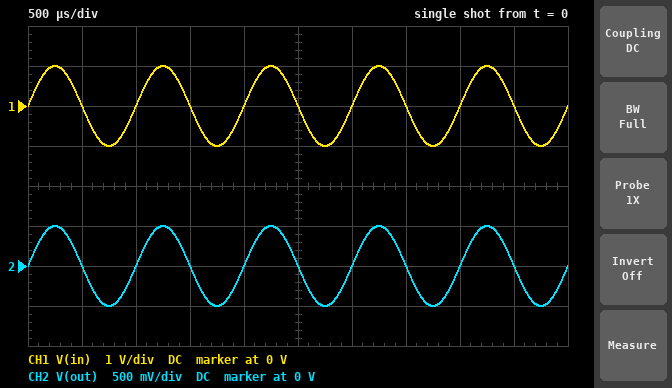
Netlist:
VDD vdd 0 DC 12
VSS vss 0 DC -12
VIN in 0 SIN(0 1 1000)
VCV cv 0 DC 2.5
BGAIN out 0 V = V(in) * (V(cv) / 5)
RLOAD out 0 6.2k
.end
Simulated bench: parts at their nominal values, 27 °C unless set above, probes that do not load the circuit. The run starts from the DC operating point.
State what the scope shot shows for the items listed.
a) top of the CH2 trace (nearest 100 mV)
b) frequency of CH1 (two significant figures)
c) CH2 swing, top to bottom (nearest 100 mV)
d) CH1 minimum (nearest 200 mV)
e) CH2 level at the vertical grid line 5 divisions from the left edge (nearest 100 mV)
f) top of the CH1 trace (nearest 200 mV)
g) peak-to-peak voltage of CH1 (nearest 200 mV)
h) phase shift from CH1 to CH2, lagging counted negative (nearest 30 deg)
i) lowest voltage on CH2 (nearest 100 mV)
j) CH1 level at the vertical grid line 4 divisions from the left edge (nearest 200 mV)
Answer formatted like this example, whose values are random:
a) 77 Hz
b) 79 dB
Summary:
a) 500 mV
b) 1.0 kHz
c) 1.0 V
d) -1.0 V
e) 0 V
f) 1.0 V
g) 2.0 V
h) 0 deg
i) -500 mV
j) 0 V
